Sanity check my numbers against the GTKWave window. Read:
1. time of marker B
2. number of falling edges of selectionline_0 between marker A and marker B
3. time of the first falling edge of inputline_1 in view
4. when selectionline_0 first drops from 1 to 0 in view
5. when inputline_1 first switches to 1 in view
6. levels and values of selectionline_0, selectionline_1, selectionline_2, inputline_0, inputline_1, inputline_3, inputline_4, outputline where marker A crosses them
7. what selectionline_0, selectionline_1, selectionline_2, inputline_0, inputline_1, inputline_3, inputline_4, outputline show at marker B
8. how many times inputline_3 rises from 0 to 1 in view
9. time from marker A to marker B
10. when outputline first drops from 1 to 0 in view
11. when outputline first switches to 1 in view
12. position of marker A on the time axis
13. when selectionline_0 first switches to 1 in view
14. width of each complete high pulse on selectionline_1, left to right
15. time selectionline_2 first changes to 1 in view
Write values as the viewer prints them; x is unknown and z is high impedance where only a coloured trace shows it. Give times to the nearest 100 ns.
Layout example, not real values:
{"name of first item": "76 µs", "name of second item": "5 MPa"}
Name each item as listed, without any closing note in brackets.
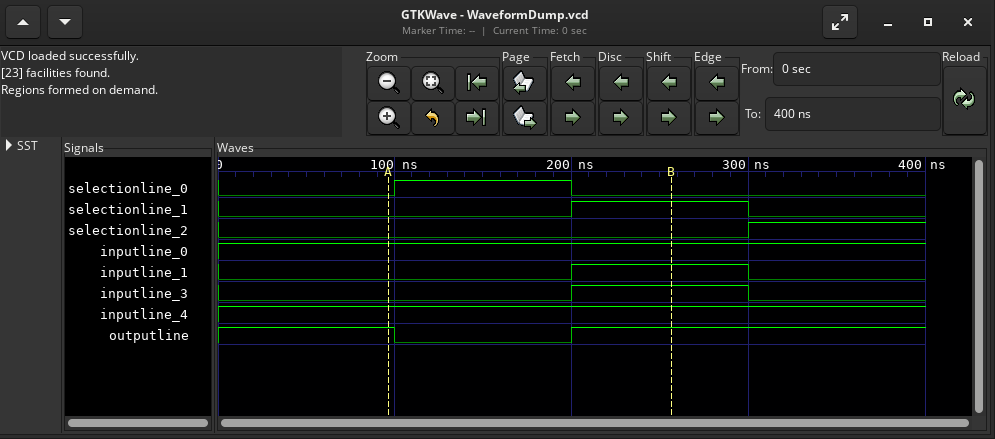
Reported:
{"time of marker B": "300 ns", "number of falling edges of selectionline_0 between marker A and marker B": "1", "time of the first falling edge of inputline_1 in view": "300 ns", "when selectionline_0 first drops from 1 to 0 in view": "200 ns", "when inputline_1 first switches to 1 in view": "200 ns", "levels and values of selectionline_0, selectionline_1, selectionline_2, inputline_0, inputline_1, inputline_3, inputline_4, outputline where marker A crosses them": "selectionline_0=0, selectionline_1=0, selectionline_2=0, inputline_0=1, inputline_1=0, inputline_3=0, inputline_4=1, outputline=1", "what selectionline_0, selectionline_1, selectionline_2, inputline_0, inputline_1, inputline_3, inputline_4, outputline show at marker B": "selectionline_0=0, selectionline_1=1, selectionline_2=0, inputline_0=1, inputline_1=1, inputline_3=1, inputline_4=1, outputline=1", "how many times inputline_3 rises from 0 to 1 in view": "1", "time from marker A to marker B": "200 ns", "when outputline first drops from 1 to 0 in view": "100 ns", "when outputline first switches to 1 in view": "200 ns", "position of marker A on the time axis": "100 ns", "when selectionline_0 first switches to 1 in view": "100 ns", "width of each complete high pulse on selectionline_1, left to right": "100 ns", "time selectionline_2 first changes to 1 in view": "300 ns"}
